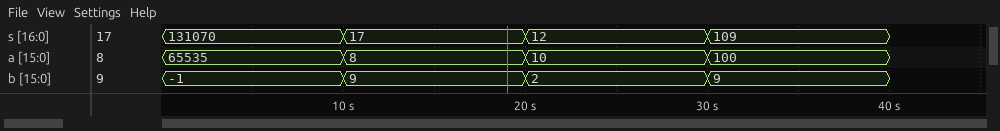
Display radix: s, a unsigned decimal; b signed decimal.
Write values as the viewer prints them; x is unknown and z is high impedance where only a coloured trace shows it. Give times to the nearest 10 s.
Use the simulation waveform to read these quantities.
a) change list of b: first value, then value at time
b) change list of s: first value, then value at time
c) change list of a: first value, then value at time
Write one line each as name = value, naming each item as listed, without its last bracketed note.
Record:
change list of b: first value, then value at time = -1, 9 at 10 s, 2 at 20 s, 9 at 30 s
change list of s: first value, then value at time = 131070, 17 at 10 s, 12 at 20 s, 109 at 30 s
change list of a: first value, then value at time = 65535, 8 at 10 s, 10 at 20 s, 100 at 30 s
